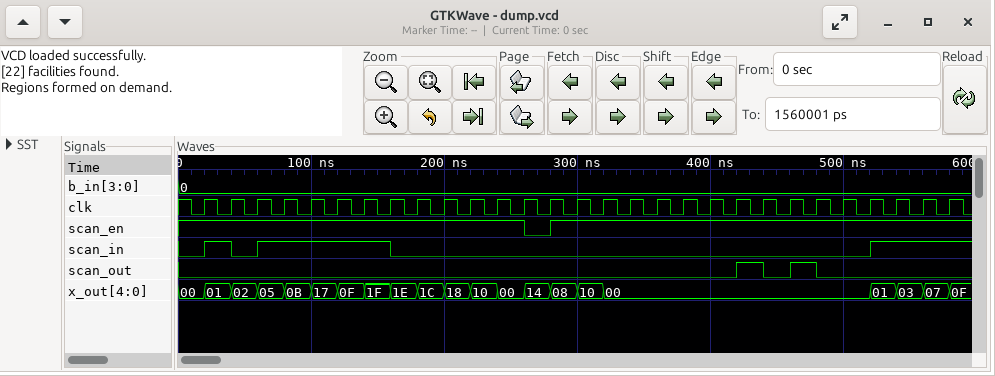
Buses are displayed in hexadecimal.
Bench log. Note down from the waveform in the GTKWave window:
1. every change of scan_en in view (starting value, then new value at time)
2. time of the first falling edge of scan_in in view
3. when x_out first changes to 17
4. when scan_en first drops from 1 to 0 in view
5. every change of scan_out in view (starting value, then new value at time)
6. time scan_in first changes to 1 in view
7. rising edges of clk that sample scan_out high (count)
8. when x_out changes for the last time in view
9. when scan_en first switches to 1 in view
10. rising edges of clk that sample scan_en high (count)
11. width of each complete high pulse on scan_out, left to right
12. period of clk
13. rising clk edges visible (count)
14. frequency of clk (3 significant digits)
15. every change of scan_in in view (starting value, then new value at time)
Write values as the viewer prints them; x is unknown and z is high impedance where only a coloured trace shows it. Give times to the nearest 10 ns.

1, 0 at 260 ns, 1 at 280 ns
40 ns
100 ns
260 ns
0, 1 at 420 ns, 0 at 440 ns, 1 at 460 ns, 0 at 480 ns
20 ns
2
580 ns
280 ns
28
20 ns, 20 ns
20 ns
29
50.0 MHz
0, 1 at 20 ns, 0 at 40 ns, 1 at 60 ns, 0 at 160 ns, 1 at 520 ns
